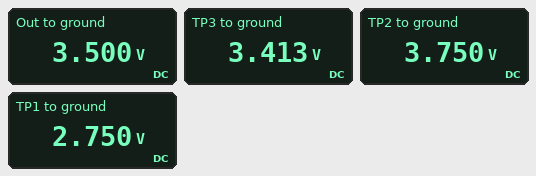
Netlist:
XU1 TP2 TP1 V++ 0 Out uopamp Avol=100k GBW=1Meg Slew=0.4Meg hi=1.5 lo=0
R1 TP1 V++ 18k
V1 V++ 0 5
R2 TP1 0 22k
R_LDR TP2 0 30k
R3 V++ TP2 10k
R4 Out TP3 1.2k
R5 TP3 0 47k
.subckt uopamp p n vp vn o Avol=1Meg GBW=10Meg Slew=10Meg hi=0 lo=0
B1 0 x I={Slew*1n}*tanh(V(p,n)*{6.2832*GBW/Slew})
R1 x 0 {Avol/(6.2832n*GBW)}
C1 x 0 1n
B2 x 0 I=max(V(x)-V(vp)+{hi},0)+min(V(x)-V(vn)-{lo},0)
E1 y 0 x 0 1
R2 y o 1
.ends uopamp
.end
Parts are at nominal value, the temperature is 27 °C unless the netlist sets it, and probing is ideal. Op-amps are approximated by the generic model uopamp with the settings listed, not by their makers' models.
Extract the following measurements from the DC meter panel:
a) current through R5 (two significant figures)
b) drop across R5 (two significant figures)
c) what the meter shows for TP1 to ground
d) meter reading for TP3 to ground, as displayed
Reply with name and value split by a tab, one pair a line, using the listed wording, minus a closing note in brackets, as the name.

current through R5	73 µA
drop across R5	3.4 V
what the meter shows for TP1 to ground	2.750 V
meter reading for TP3 to ground, as displayed	3.413 V
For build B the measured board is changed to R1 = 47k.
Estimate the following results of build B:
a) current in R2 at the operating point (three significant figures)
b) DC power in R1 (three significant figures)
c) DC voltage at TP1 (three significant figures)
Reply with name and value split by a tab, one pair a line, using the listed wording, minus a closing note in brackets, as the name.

current in R2 at the operating point	72.5 µA
DC power in R1	247 µW
DC voltage at TP1	1.59 V
